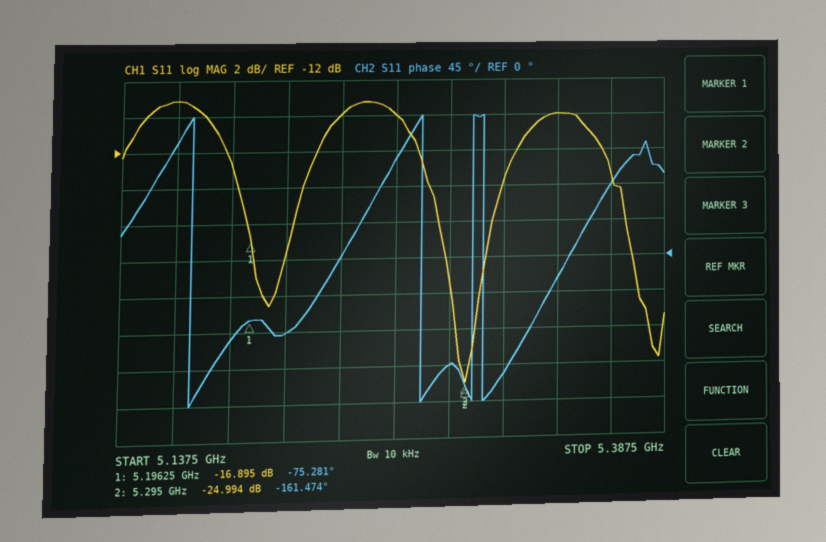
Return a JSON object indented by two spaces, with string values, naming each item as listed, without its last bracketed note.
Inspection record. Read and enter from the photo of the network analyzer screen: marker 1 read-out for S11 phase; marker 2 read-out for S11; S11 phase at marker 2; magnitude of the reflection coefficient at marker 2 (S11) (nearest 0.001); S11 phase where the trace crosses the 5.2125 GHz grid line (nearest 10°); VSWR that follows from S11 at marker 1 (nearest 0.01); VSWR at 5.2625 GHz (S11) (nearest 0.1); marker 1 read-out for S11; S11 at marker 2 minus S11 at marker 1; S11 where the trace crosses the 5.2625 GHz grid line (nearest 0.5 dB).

{
  "marker 1 read-out for S11 phase": "-75.281°",
  "marker 2 read-out for S11": "-24.994 dB",
  "S11 phase at marker 2": "-161.474°",
  "magnitude of the reflection coefficient at marker 2 (S11)": "0.056",
  "S11 phase where the trace crosses the 5.2125 GHz grid line": "-90°",
  "VSWR that follows from S11 at marker 1": "1.33",
  "VSWR at 5.2625 GHz (S11)": "1.9",
  "marker 1 read-out for S11": "-16.895 dB",
  "S11 at marker 2 minus S11 at marker 1": "-8.099 dB",
  "S11 where the trace crosses the 5.2625 GHz grid line": "-10.0 dB"
}
